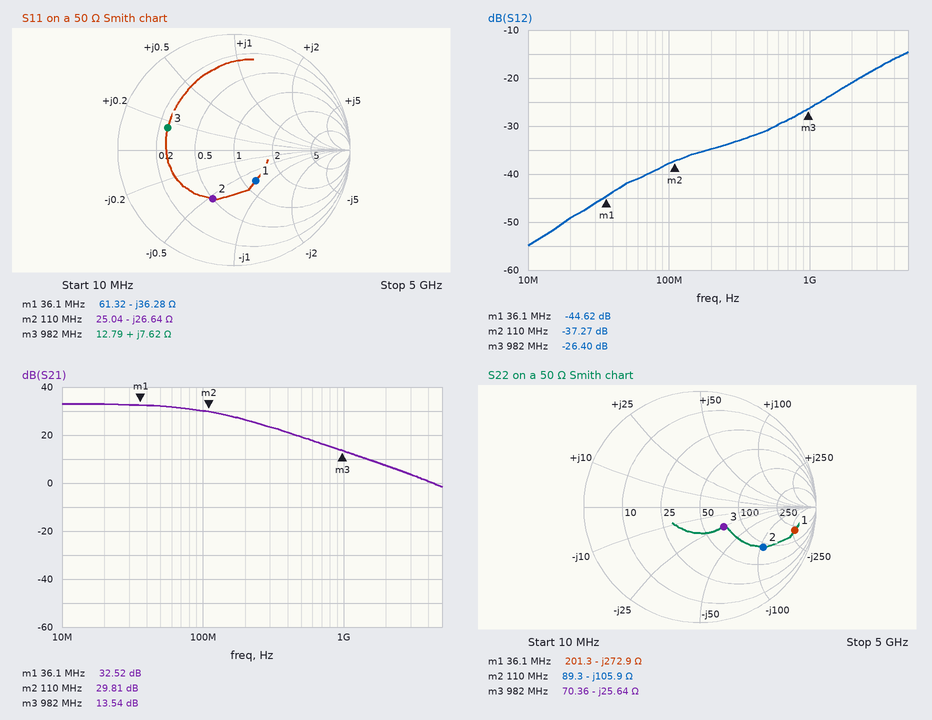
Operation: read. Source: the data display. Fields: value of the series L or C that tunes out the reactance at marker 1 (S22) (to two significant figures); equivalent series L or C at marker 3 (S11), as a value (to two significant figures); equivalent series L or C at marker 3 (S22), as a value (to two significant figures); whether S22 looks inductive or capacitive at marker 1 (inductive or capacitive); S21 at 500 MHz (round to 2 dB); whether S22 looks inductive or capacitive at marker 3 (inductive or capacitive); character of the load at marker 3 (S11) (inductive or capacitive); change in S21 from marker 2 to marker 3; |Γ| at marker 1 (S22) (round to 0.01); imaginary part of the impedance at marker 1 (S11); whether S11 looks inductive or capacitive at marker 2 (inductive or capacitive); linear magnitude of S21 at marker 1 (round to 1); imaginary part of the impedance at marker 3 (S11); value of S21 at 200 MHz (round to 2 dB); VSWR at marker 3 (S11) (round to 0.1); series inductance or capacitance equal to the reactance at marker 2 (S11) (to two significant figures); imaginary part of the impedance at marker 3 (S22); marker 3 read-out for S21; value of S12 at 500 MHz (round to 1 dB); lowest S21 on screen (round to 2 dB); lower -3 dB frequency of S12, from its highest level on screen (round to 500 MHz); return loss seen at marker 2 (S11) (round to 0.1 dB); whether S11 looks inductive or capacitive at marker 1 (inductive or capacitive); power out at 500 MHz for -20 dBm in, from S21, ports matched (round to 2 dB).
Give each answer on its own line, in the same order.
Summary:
1.2 µH
1.2 nH
6.3 pF
capacitive
20 dB
capacitive
inductive
-16.27 dB
0.84
-36.28 Ω
capacitive
42
+7.62 Ω
26 dB
4.0
54 pF
-25.64 Ω
13.54 dB
-31 dB
-2 dB
3.0 GHz
6.8 dB
capacitive
0 dBm
